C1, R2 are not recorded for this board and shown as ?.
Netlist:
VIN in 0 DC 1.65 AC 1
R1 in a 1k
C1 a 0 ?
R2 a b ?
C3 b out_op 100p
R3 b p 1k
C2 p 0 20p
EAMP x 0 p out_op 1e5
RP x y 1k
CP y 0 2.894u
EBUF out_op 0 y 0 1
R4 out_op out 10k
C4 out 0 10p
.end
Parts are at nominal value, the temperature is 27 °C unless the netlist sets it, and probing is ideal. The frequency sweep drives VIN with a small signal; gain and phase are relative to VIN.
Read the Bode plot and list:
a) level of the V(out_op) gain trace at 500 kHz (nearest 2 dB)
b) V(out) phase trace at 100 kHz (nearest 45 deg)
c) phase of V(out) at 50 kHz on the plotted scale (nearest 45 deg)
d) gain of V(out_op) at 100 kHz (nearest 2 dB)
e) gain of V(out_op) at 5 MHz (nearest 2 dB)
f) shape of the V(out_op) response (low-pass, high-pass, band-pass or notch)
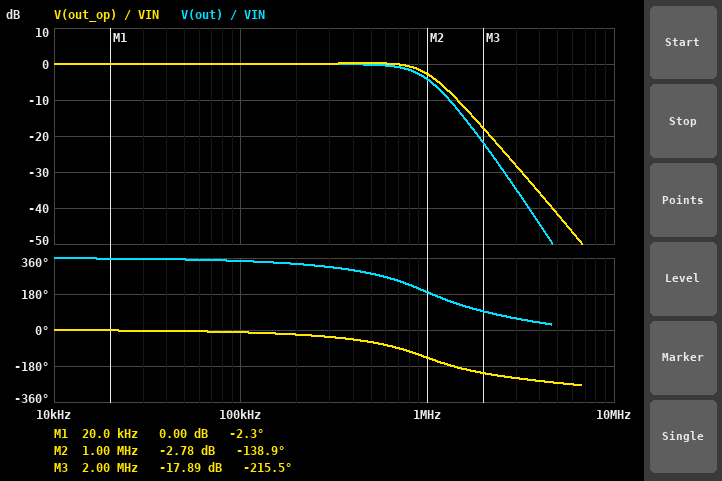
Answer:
0 dB
360 deg
360 deg
0 dB
-42 dB
low-pass
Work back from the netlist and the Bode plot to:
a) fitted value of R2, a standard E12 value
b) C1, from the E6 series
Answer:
4.7 kΩ
150 pF
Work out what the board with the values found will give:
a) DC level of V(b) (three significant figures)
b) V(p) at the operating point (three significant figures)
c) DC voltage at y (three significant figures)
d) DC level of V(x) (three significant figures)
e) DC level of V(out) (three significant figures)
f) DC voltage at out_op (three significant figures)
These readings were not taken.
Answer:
1.65 V
1.65 V
1.65 V
1.65 V
1.65 V
1.65 V
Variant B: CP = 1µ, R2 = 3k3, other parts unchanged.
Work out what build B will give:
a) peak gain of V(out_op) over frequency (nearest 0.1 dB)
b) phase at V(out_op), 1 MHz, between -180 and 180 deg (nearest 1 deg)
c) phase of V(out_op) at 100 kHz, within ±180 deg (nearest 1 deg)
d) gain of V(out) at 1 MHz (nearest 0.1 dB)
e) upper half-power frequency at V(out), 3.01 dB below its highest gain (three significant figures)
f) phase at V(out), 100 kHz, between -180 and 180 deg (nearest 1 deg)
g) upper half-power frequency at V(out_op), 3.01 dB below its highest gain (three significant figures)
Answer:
0 dB
-95 deg
-10 deg
-3.4 dB
936 kHz
-13 deg
1.21 MHz
